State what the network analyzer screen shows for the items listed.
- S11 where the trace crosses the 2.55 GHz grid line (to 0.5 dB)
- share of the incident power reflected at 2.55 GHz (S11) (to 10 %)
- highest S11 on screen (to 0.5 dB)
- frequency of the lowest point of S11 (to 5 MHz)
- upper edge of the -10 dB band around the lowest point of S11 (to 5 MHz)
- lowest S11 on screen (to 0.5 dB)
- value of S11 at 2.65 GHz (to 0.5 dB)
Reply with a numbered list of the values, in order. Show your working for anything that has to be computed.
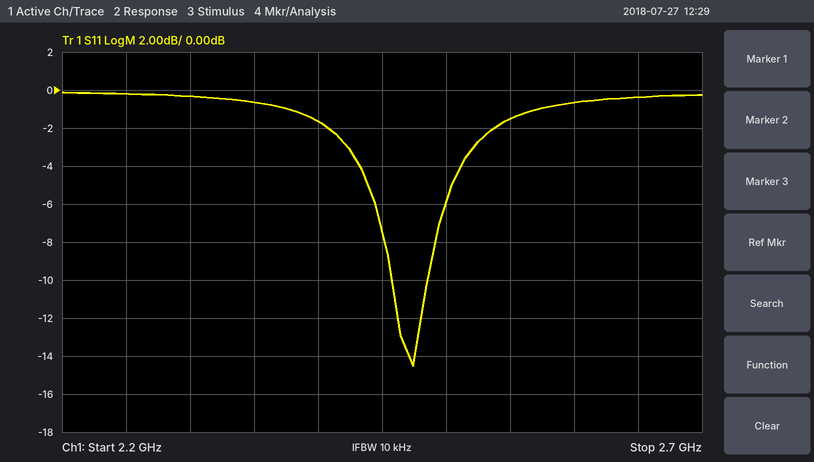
1. -1.5 dB
2. 10^(-1.5/10) ≈ 70.8 %, so 70 % to the nearest 10 %
3. 0.0 dB
4. 2.475 GHz
5. 2.485 GHz
6. -14.5 dB
7. -0.5 dB
